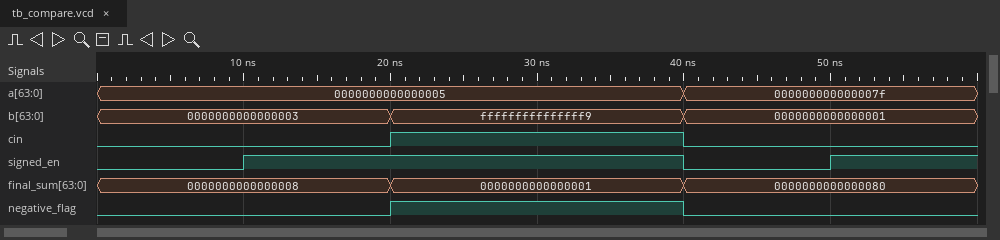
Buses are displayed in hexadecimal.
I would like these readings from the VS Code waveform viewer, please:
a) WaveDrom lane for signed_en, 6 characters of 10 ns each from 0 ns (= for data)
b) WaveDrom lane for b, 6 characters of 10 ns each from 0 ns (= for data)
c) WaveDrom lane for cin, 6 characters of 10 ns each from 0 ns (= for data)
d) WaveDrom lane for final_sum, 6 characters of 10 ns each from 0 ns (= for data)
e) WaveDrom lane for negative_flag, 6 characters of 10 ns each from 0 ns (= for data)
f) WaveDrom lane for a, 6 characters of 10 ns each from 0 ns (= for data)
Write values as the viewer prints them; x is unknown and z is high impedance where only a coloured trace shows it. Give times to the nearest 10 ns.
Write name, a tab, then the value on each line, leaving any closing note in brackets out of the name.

WaveDrom lane for signed_en, 6 characters of 10 ns each from 0 ns	{name: 'signed_en', wave: '01..01'}
WaveDrom lane for b, 6 characters of 10 ns each from 0 ns	{name: 'b', wave: '=.=.=.', data: '0000000000000003 fffffffffffffff9 0000000000000001'}
WaveDrom lane for cin, 6 characters of 10 ns each from 0 ns	{name: 'cin', wave: '0.1.0.'}
WaveDrom lane for final_sum, 6 characters of 10 ns each from 0 ns	{name: 'final_sum', wave: '=.=.=.', data: '0000000000000008 0000000000000001 0000000000000080'}
WaveDrom lane for negative_flag, 6 characters of 10 ns each from 0 ns	{name: 'negative_flag', wave: '0.1.0.'}
WaveDrom lane for a, 6 characters of 10 ns each from 0 ns	{name: 'a', wave: '=...=.', data: '0000000000000005 000000000000007f'}
